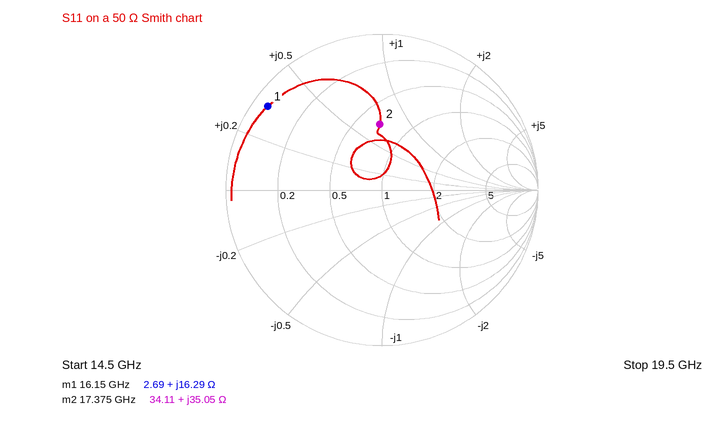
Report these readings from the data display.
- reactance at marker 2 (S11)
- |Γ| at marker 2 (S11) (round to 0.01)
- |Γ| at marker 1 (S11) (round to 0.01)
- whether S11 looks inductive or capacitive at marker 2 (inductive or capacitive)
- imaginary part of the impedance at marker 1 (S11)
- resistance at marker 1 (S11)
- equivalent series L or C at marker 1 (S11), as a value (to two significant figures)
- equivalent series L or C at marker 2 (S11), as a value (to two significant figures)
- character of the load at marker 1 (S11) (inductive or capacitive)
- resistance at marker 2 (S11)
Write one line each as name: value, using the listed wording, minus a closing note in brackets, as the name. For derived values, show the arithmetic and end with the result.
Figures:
reactance at marker 2: +35.05 Ω
|Γ| at marker 2 (S11): 0.42
|Γ| at marker 1 (S11): 0.91
whether S11 looks inductive or capacitive at marker 2: inductive
imaginary part of the impedance at marker 1: +16.29 Ω
resistance at marker 1: 2.69 Ω
equivalent series L or C at marker 1 (S11), as a value: L = 16.29 Ω/(2π × 16.15 GHz) ≈ 161 pH, so 160 pH to two significant figures
equivalent series L or C at marker 2 (S11), as a value: L = 35.05 Ω/(2π × 17.375 GHz) ≈ 321 pH, so 320 pH to two significant figures
character of the load at marker 1 (S11): inductive
resistance at marker 2: 34.11 Ω
